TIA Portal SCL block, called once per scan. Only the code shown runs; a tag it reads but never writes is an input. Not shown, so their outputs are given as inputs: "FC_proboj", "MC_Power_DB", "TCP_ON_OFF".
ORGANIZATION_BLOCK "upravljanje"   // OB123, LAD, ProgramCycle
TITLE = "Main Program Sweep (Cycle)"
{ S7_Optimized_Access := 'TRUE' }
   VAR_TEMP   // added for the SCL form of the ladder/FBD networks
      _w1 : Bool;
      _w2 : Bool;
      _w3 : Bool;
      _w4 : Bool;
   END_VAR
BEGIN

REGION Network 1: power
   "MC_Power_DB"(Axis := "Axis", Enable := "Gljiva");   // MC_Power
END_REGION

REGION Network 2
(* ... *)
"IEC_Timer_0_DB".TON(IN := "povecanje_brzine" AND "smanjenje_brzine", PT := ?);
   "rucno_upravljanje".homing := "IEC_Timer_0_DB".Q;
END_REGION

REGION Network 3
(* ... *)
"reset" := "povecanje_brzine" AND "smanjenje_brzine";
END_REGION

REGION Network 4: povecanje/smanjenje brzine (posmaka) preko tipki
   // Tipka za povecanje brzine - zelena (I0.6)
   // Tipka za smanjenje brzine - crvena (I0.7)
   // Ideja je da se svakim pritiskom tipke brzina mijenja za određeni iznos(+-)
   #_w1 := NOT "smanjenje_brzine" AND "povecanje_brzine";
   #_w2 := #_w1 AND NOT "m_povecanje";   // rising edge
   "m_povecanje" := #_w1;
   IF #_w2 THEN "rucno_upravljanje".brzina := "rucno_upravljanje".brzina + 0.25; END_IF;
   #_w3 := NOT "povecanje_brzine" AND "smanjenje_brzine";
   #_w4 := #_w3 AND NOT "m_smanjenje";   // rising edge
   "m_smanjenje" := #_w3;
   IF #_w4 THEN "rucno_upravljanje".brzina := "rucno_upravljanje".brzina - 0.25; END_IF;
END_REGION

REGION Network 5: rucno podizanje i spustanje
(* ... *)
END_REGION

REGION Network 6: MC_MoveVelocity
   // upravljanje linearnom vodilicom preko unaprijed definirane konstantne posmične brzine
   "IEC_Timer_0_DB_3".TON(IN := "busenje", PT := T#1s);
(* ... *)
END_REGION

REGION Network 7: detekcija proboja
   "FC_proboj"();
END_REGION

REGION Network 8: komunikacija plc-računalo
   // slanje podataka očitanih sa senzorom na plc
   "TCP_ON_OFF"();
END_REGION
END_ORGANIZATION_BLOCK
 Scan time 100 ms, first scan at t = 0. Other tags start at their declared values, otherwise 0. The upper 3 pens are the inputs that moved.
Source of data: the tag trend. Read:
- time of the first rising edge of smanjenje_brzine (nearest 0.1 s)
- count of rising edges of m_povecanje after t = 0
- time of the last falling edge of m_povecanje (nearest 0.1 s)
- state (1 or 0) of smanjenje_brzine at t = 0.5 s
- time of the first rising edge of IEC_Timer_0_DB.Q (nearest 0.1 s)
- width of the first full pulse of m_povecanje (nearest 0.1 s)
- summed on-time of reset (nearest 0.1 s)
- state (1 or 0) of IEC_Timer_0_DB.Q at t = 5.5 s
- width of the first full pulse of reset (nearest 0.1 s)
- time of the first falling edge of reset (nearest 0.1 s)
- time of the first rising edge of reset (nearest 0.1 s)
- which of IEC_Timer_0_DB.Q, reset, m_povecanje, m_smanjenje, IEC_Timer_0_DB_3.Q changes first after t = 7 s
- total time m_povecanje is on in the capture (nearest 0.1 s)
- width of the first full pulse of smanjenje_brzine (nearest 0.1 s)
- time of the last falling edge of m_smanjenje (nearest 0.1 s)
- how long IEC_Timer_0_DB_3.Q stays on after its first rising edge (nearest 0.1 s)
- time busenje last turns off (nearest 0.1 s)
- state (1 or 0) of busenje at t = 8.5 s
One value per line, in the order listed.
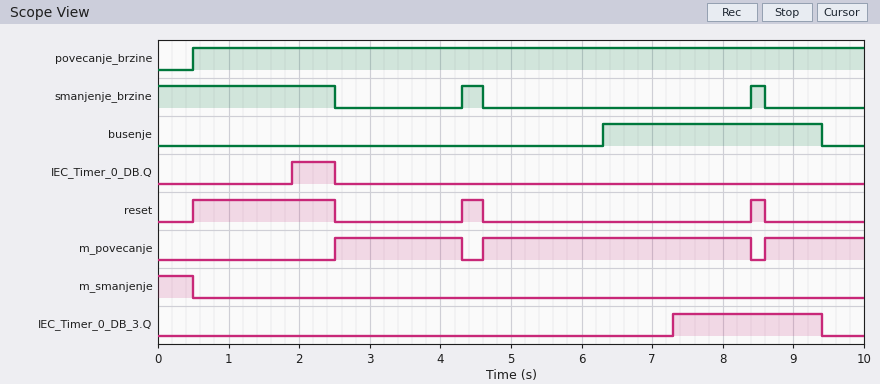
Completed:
4.3 s
3
8.4 s
1
1.9 s
1.8 s
2.5 s
0
2.0 s
2.5 s
0.5 s
IEC_Timer_0_DB_3.Q
7.0 s
0.3 s
0.5 s
2.1 s
9.4 s
1
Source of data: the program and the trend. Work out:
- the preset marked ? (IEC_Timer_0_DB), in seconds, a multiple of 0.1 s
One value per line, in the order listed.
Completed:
1.4 s
